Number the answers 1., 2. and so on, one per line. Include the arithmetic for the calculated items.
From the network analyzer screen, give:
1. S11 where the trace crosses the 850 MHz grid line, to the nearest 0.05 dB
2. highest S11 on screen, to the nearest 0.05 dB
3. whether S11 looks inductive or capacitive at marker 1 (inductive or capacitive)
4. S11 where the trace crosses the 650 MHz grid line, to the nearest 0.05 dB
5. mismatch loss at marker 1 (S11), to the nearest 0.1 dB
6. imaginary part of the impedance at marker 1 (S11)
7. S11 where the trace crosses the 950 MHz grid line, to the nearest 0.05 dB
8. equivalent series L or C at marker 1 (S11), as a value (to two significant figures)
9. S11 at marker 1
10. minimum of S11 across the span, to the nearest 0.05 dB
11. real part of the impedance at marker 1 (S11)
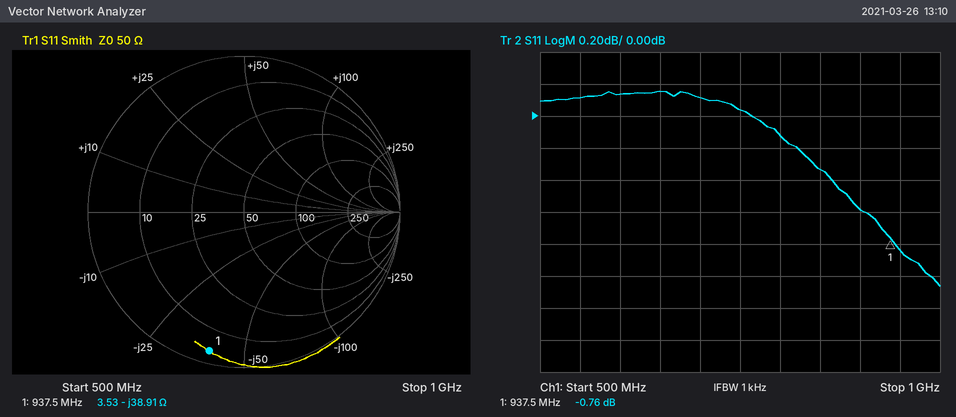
1. -0.35 dB
2. 0.15 dB
3. capacitive
4. 0.15 dB
5. −10 log10(1 − 10^(-0.76/10)) ≈ 7.9 dB
6. -38.91 Ω
7. -0.85 dB
8. C = 1/(2π × 937.5 MHz × 38.91 Ω) ≈ 4.4 pF
9. -0.76 dB
10. -1.05 dB
11. 3.53 Ω
